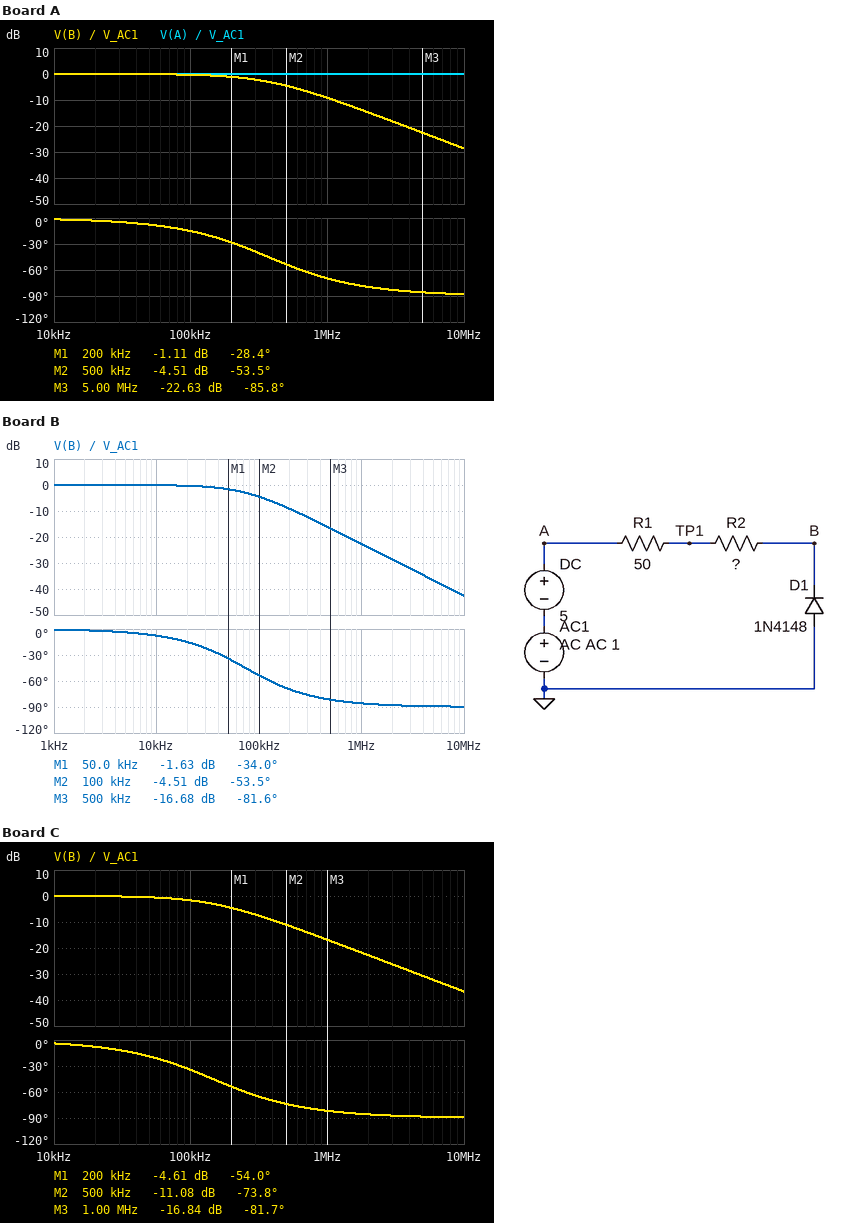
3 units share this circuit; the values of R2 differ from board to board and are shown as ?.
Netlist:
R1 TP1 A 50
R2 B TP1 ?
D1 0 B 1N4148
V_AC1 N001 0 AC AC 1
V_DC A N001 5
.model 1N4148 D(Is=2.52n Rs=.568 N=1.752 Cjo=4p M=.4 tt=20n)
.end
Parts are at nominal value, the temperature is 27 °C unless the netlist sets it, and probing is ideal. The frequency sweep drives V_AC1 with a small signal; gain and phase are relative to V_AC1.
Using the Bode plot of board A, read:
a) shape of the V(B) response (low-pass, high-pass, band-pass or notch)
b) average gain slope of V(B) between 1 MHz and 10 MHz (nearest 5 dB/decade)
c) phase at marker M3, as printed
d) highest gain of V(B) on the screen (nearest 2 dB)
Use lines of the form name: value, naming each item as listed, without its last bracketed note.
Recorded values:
shape of the V(B) response: low-pass
average gain slope of V(B) between 1 MHz and 10 MHz: -20 dB/decade
phase at marker M3, as printed: -85.8 deg
highest gain of V(B) on the screen: 0 dB
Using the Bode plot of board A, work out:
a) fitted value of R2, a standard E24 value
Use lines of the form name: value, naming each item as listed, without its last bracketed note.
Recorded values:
fitted value of R2, a standard E24 value: 220 kΩ
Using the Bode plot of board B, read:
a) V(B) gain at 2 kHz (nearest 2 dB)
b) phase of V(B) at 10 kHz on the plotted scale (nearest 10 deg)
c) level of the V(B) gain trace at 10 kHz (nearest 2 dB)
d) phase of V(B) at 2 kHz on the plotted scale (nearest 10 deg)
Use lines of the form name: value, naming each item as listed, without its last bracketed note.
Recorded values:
V(B) gain at 2 kHz: 0 dB
phase of V(B) at 10 kHz on the plotted scale: -10 deg
level of the V(B) gain trace at 10 kHz: 0 dB
phase of V(B) at 2 kHz on the plotted scale: 0 deg
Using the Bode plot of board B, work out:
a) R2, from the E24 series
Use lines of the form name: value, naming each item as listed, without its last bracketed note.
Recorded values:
R2, from the E24 series: 1.1 MΩ
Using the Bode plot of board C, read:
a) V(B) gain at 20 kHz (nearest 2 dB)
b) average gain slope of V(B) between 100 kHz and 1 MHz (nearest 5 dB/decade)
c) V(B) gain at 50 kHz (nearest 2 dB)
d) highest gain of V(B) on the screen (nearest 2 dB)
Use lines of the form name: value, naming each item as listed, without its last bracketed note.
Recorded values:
V(B) gain at 20 kHz: 0 dB
average gain slope of V(B) between 100 kHz and 1 MHz: -15 dB/decade
V(B) gain at 50 kHz: 0 dB
highest gain of V(B) on the screen: 0 dB
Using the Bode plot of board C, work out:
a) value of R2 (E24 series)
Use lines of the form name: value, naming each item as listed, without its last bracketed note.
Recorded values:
value of R2: 560 kΩ
